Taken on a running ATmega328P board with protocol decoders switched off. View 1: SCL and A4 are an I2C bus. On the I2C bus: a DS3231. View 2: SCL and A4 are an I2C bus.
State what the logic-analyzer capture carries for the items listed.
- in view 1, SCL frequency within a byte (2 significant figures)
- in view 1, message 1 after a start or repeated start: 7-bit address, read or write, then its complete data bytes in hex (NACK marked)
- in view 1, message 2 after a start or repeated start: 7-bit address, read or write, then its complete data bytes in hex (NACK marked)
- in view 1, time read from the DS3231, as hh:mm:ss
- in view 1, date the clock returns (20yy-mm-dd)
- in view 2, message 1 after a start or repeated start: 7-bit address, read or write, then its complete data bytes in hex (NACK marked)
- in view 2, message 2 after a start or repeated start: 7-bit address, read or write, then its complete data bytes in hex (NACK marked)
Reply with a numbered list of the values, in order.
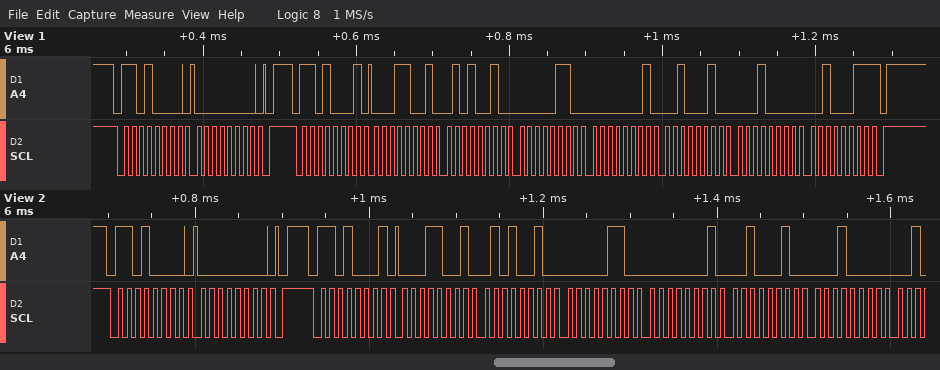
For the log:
1. 100 kHz
2. 0x68 write: 00
3. 0x68 read: 19 52 06 01 22 10 23 NACK
4. 06:52:19
5. 2023-10-22
6. 0x68 write: 00
7. 0x68 read: 19 52 06 01 22 10
